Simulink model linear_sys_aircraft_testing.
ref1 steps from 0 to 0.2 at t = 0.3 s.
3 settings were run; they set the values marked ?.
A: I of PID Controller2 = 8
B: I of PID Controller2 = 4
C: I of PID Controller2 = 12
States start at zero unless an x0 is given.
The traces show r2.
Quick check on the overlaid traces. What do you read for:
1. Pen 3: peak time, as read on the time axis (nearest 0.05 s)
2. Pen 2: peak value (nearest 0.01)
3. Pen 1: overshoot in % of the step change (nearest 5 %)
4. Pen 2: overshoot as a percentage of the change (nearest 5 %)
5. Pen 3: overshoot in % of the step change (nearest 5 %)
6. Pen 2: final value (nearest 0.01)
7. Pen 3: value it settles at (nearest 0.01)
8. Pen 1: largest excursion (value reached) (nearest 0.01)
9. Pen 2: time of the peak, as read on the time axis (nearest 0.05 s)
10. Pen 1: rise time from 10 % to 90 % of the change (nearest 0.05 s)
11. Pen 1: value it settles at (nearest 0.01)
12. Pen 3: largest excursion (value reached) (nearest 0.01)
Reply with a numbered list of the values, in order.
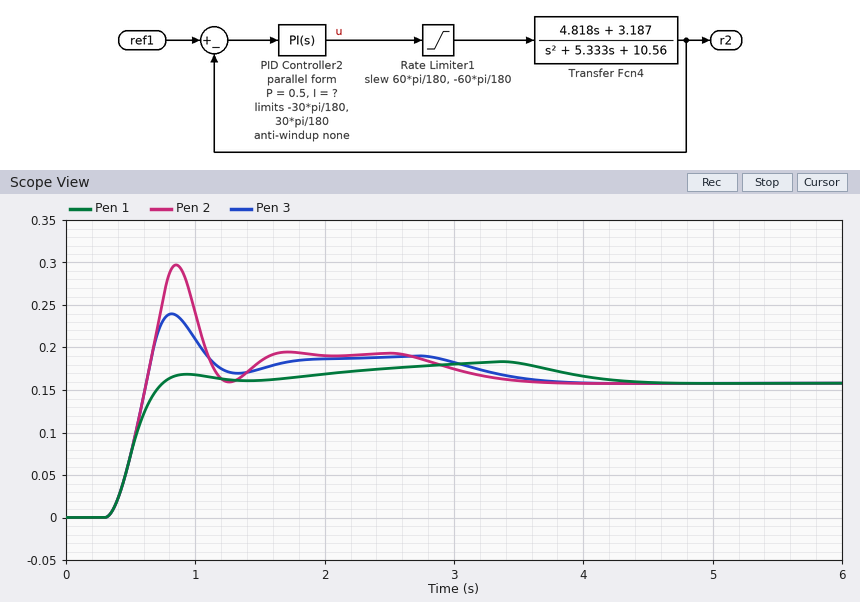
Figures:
1. 0.80 s
2. 0.30
3. 15 %
4. 90 %
5. 50 %
6. 0.16
7. 0.16
8. 0.18
9. 0.85 s
10. 0.30 s
11. 0.16
12. 0.24
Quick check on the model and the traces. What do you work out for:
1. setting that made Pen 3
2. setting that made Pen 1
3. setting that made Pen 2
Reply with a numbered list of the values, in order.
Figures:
1. A
2. B
3. C
